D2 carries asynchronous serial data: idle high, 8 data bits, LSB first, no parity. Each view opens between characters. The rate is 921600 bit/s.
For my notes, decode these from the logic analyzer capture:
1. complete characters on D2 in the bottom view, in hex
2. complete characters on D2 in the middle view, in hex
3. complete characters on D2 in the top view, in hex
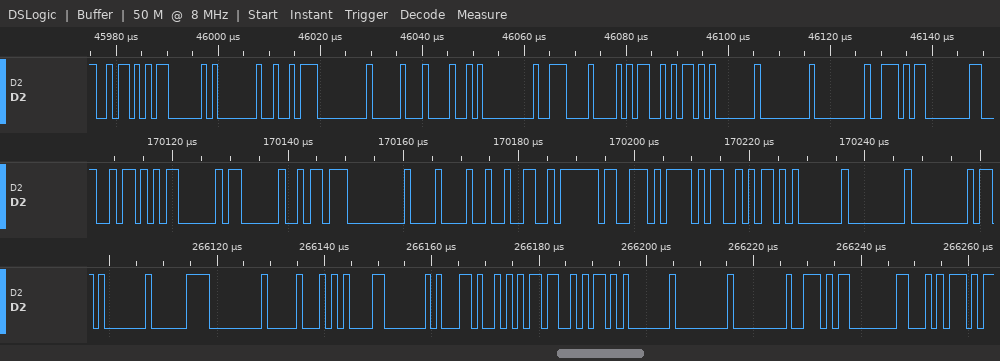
01, E0, 00, 10, 85, 40, 2C, B5, 6A, 01, 00, 00, AE, 80, D4
5A, 03, 03, DA, 00, 08, 92, FA, 73, AF, 6A, 01, 00, 00
5A, 03, 01, D2, 00, 10, 48, 00, 0E, A8, 6A, 01, 00, 00, AE, 80
